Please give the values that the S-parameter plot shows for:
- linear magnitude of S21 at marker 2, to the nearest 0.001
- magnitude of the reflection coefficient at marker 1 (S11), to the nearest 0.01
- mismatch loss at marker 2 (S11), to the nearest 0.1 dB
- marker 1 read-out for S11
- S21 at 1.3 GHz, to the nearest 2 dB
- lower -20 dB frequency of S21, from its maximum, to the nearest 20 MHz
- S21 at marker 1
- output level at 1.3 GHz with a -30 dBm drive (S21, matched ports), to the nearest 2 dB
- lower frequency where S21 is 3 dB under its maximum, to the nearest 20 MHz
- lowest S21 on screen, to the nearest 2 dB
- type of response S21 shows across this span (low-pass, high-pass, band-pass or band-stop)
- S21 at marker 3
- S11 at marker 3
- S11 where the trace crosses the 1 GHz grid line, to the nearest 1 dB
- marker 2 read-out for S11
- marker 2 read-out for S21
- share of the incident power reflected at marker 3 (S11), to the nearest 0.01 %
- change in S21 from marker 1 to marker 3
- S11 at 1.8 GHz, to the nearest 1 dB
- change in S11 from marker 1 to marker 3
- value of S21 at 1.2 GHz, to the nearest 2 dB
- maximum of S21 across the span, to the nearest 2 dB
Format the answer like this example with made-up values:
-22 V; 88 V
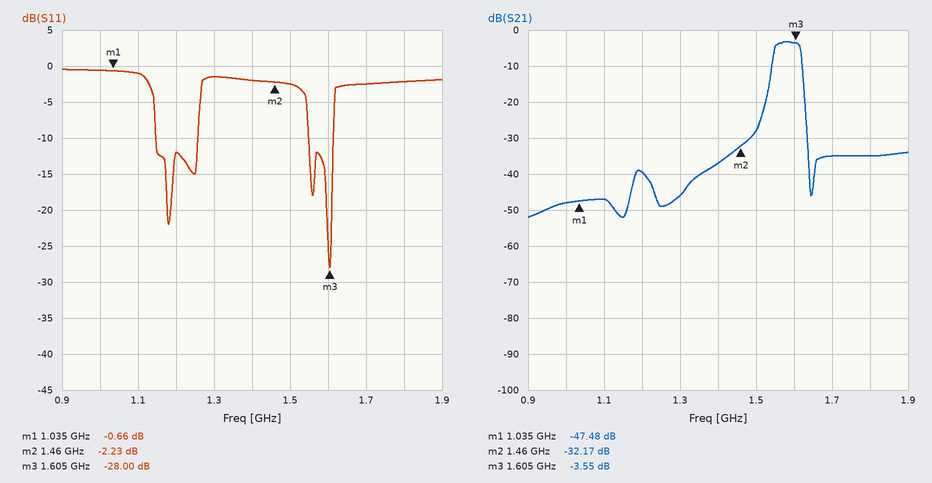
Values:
0.025; 0.93; 4.0 dB; -0.66 dB; -46 dB; 1.52 GHz; -47.48 dB; -76 dBm; 1.54 GHz; -52 dB; band-pass; -3.55 dB; -28.00 dB; -1 dB; -2.23 dB; -32.17 dB; 0.16 %; 43.93 dB; -2 dB; -27.34 dB; -40 dB; -4 dB
